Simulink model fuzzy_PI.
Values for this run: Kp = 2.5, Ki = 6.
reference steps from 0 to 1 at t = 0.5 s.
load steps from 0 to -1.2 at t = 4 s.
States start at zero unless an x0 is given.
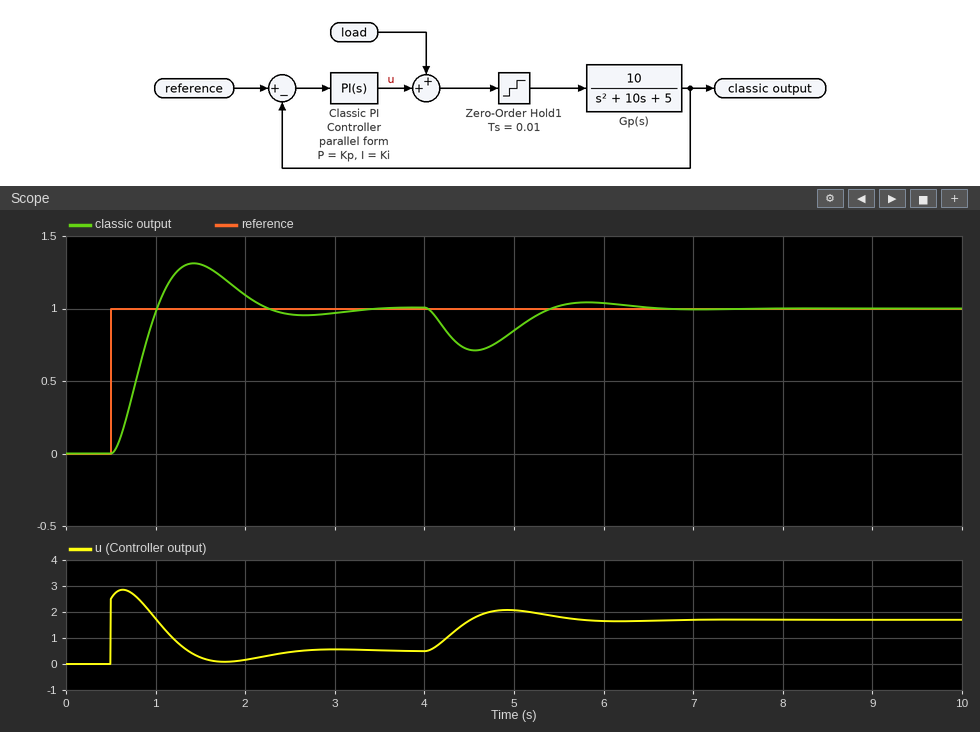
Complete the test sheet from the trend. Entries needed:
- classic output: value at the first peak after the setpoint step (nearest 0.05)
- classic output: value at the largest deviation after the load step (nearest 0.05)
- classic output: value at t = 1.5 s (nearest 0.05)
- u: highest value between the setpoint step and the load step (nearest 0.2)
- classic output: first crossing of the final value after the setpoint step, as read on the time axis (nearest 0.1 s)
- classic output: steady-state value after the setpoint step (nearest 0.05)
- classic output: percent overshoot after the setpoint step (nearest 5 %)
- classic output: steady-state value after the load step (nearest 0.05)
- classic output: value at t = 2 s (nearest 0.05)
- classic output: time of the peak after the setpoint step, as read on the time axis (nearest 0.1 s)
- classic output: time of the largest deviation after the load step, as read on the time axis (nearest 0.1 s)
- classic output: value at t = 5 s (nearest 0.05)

1.30
0.70
1.30
2.8
1.0 s
1.00
30 %
1.00
1.10
1.4 s
4.6 s
0.85
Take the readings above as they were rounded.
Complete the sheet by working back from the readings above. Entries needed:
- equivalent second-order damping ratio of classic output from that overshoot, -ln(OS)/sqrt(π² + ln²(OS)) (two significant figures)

0.36
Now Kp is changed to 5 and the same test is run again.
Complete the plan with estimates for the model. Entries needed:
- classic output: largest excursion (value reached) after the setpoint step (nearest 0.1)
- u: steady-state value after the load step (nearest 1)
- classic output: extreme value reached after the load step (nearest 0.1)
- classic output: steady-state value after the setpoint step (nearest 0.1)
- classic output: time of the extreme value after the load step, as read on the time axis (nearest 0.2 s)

1.2
2
0.8
1.0
4.4 s
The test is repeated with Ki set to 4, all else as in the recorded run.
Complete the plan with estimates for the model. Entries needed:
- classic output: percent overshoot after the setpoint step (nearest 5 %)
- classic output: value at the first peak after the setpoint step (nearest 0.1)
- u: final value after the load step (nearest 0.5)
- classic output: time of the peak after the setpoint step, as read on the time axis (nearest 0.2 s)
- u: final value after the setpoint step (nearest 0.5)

20 %
1.2
1.5
1.6 s
0.5
